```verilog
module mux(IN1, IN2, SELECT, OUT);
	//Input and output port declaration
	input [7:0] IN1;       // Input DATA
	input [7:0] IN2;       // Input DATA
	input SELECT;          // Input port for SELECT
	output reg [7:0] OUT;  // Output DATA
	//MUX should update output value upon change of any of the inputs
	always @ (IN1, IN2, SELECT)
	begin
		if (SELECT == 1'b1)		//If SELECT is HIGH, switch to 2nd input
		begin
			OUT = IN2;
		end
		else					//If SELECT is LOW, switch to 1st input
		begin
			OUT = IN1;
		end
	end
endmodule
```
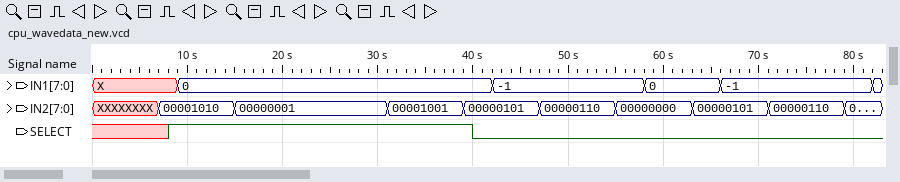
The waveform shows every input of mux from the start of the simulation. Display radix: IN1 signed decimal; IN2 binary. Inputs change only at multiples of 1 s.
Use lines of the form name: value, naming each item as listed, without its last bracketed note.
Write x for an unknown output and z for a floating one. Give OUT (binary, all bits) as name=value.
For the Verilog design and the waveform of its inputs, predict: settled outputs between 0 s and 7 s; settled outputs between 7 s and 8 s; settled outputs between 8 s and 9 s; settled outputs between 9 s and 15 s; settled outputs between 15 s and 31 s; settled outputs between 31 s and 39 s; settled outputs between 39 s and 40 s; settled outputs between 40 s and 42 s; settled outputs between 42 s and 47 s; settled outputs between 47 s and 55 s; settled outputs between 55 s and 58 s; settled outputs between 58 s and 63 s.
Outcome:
settled outputs between 0 s and 7 s: OUT=x
settled outputs between 7 s and 8 s: OUT=x
settled outputs between 8 s and 9 s: OUT=00001010
settled outputs between 9 s and 15 s: OUT=00001010
settled outputs between 15 s and 31 s: OUT=00000001
settled outputs between 31 s and 39 s: OUT=00001001
settled outputs between 39 s and 40 s: OUT=00000101
settled outputs between 40 s and 42 s: OUT=00000000
settled outputs between 42 s and 47 s: OUT=11111111
settled outputs between 47 s and 55 s: OUT=11111111
settled outputs between 55 s and 58 s: OUT=11111111
settled outputs between 58 s and 63 s: OUT=00000000
